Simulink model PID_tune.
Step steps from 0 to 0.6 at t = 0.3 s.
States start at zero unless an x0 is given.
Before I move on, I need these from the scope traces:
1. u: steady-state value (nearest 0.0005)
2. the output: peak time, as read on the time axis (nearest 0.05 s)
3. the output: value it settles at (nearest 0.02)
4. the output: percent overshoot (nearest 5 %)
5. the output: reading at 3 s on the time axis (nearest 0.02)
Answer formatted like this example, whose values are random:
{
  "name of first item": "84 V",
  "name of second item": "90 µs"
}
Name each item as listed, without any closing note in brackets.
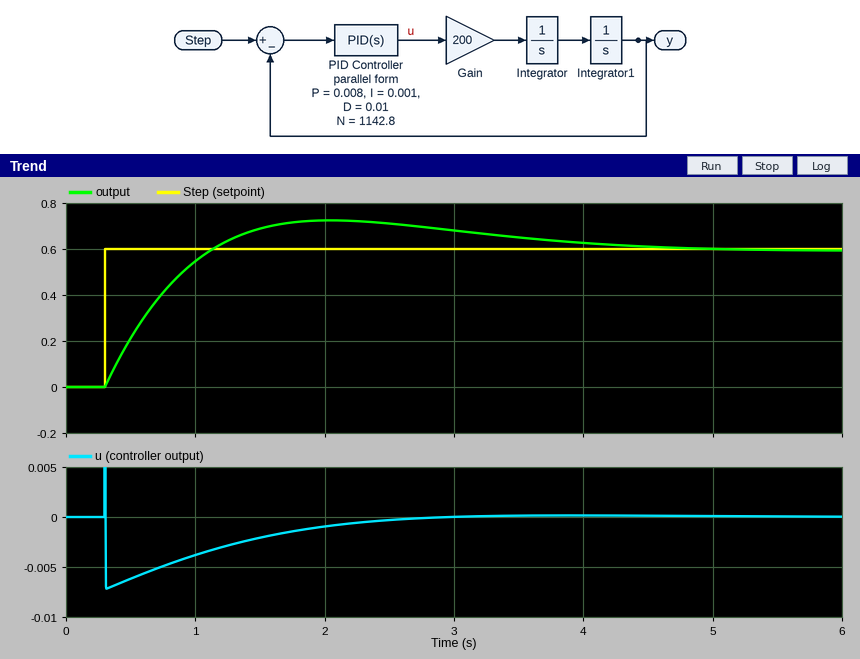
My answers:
{
  "u: steady-state value": "0.0000",
  "the output: peak time, as read on the time axis": "2.05 s",
  "the output: value it settles at": "0.60",
  "the output: percent overshoot": "20 %",
  "the output: reading at 3 s on the time axis": "0.68"
}
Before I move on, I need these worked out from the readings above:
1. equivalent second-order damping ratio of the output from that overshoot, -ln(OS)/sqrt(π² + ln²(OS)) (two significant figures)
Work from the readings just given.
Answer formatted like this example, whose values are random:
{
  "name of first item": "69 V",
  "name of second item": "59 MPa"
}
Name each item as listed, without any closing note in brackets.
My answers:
{
  "equivalent second-order damping ratio of the output from that overshoot, -ln(OS)/sqrt(π² + ln²(OS))": "0.46"
}
